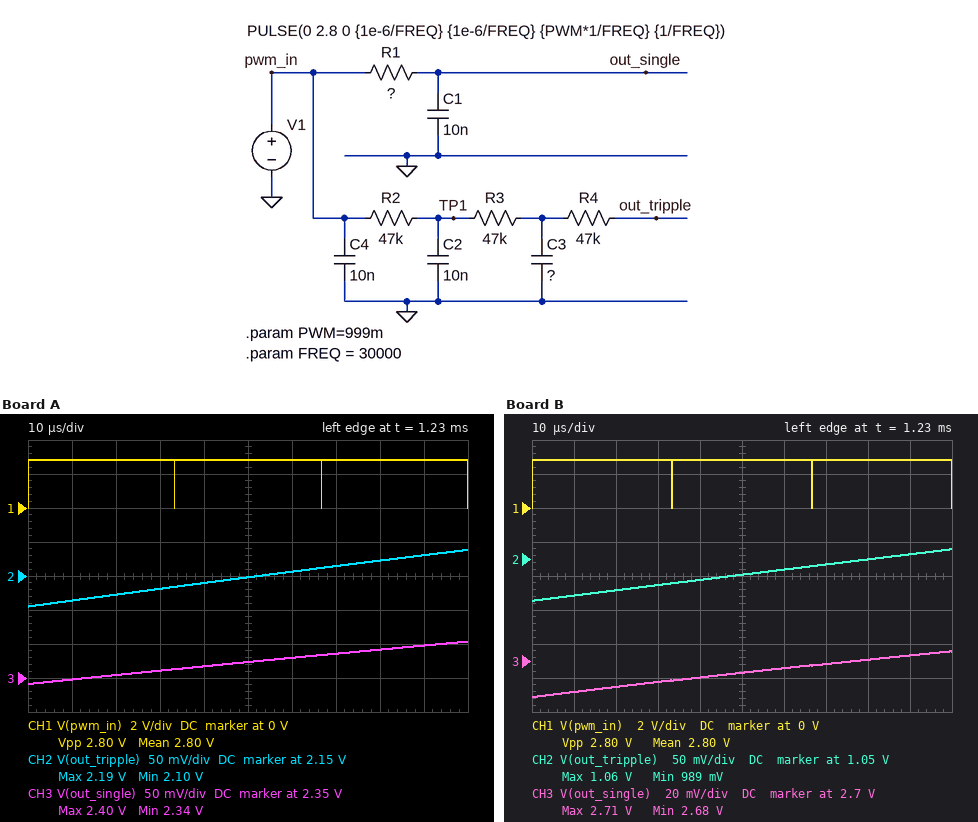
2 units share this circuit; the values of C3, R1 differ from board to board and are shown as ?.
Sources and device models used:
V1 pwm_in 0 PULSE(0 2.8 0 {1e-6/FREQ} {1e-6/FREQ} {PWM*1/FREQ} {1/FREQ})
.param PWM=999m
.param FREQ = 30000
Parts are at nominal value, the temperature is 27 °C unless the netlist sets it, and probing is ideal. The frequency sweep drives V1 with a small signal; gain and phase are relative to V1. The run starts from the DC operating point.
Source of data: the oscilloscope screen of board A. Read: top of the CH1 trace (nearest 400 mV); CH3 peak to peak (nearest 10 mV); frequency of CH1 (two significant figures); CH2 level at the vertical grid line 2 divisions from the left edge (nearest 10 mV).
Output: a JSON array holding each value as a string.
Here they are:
["2.8 V", "60 mV", "30 kHz", "2.12 V"]
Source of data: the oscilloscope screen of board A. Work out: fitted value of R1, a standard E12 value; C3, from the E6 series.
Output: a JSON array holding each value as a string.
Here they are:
["68 kΩ", "4.7 nF"]
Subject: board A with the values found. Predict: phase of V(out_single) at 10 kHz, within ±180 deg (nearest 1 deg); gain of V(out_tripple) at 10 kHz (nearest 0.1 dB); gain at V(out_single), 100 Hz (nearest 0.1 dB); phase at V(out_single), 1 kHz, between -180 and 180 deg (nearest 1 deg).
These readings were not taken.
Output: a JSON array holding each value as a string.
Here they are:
["-89 deg", "-52.3 dB", "-0.7 dB", "-77 deg"]
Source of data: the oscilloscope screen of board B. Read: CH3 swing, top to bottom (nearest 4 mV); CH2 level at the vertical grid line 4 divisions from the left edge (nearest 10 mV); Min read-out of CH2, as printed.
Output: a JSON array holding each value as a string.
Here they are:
["28 mV", "1.02 V", "989 mV"]
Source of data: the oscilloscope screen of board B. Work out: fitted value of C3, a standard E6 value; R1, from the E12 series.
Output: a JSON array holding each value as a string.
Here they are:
["22 nF", "39 kΩ"]
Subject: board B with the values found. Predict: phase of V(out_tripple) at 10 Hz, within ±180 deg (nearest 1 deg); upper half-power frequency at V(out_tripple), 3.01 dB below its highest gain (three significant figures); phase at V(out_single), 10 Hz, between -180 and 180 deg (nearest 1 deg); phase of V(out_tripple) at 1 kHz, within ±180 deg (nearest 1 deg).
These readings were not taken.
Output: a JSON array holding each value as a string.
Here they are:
["-9 deg", "67.8 Hz", "-1 deg", "-139 deg"]
